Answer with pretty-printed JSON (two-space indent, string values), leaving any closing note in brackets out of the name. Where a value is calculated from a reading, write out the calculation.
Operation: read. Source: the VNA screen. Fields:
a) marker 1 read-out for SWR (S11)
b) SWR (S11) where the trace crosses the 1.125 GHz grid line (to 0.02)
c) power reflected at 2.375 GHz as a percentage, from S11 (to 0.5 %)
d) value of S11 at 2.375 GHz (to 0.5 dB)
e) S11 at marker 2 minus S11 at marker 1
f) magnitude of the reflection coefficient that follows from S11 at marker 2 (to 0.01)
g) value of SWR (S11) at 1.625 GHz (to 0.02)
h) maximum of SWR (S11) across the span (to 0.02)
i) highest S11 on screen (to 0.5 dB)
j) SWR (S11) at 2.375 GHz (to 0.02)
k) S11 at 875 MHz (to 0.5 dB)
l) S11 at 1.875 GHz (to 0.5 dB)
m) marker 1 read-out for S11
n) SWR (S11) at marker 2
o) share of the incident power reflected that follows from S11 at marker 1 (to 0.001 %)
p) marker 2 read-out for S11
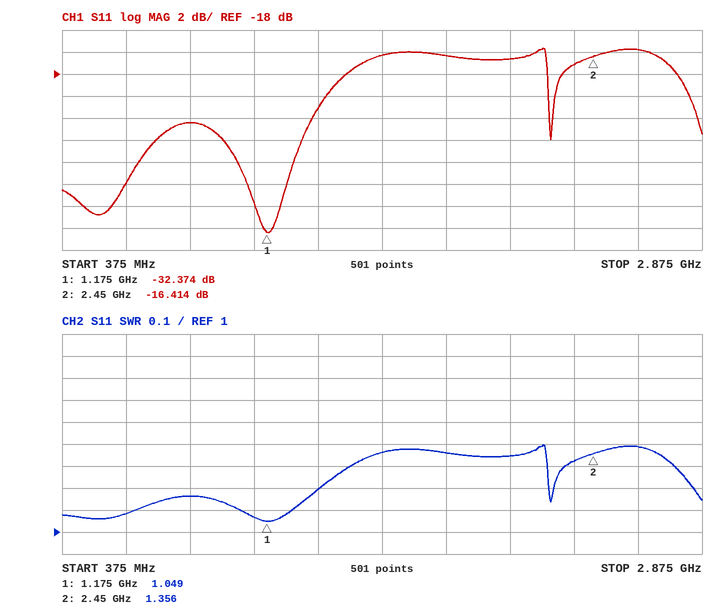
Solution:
{
  "marker 1 read-out for SWR": "1.049",
  "SWR (S11) where the trace crosses the 1.125 GHz grid line": "1.06",
  "power reflected at 2.375 GHz as a percentage, from S11": "10^(-17/10) ≈ 2.0 %",
  "value of S11 at 2.375 GHz": "-17.0 dB",
  "S11 at marker 2 minus S11 at marker 1": "-16.414 − (-32.374) = 15.960 dB",
  "magnitude of the reflection coefficient that follows from S11 at marker 2": "10^(-16.414/20) ≈ 0.15",
  "value of SWR (S11) at 1.625 GHz": "1.36",
  "maximum of SWR (S11) across the span": "1.40",
  "highest S11 on screen": "-15.5 dB",
  "SWR (S11) at 2.375 GHz": "1.32",
  "S11 at 875 MHz": "-22.5 dB",
  "S11 at 1.875 GHz": "-16.5 dB",
  "marker 1 read-out for S11": "-32.374 dB",
  "SWR (S11) at marker 2": "1.356",
  "share of the incident power reflected that follows from S11 at marker 1": "10^(-32.374/10) ≈ 0.058 %",
  "marker 2 read-out for S11": "-16.414 dB"
}
